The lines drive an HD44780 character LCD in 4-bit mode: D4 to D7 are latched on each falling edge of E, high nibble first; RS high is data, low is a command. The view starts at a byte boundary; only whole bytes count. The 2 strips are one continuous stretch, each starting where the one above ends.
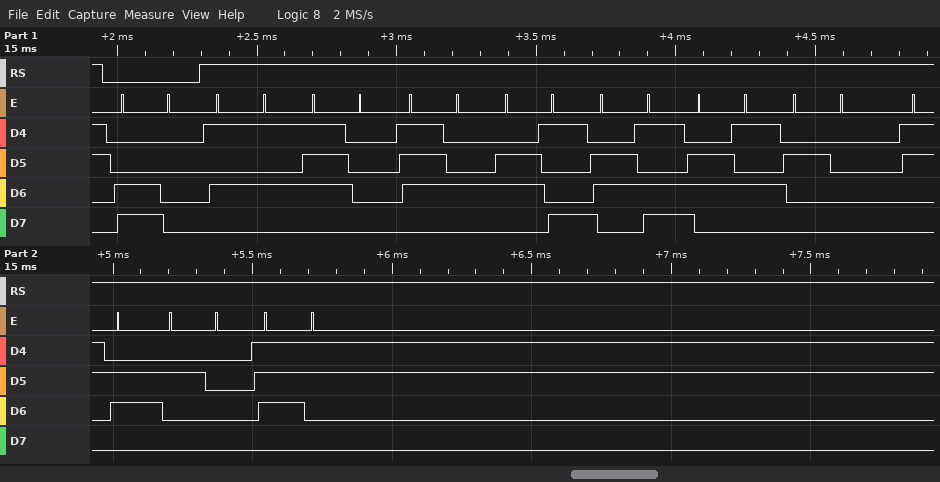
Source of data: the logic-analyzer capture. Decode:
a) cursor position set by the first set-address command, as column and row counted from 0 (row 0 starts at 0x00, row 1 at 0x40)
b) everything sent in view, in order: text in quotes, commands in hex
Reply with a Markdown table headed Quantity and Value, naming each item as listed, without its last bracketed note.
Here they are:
| Quantity | Value |
|---|---|
| cursor position set by the first set-address command, as column and row counted from 0 | column 0, row 1 |
| everything sent in view, in order: text in quotes, commands in hex | 0xC0 "Uptime 6 s" |
